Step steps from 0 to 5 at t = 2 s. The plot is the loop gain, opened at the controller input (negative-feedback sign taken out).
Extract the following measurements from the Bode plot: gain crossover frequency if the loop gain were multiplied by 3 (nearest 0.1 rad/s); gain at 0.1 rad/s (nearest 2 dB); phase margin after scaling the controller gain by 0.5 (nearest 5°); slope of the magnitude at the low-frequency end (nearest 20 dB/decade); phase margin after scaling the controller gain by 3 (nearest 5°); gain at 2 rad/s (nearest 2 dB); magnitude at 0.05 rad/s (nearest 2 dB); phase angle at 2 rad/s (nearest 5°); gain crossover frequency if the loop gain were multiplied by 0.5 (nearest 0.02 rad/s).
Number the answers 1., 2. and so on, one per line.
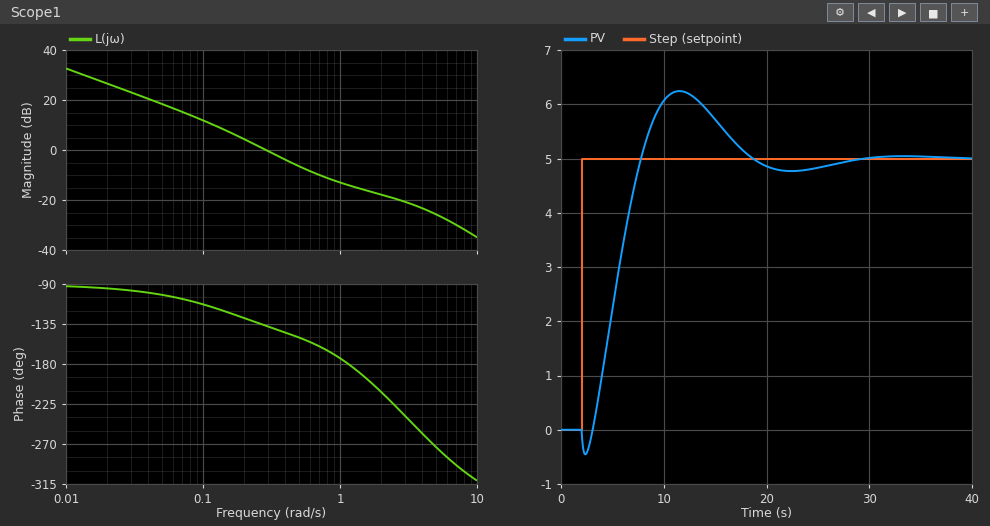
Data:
1. 0.7 rad/s
2. 12 dB
3. 55°
4. -20 dB/decade
5. 20°
6. -18 dB
7. 18 dB
8. -210°
9. 0.18 rad/s
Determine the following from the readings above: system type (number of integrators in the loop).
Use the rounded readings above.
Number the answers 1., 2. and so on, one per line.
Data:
1. 1
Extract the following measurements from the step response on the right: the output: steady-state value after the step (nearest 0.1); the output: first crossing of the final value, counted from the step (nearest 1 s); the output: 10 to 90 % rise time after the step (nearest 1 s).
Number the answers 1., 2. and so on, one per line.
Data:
1. 5.0
2. 6 s
3. 4 s
